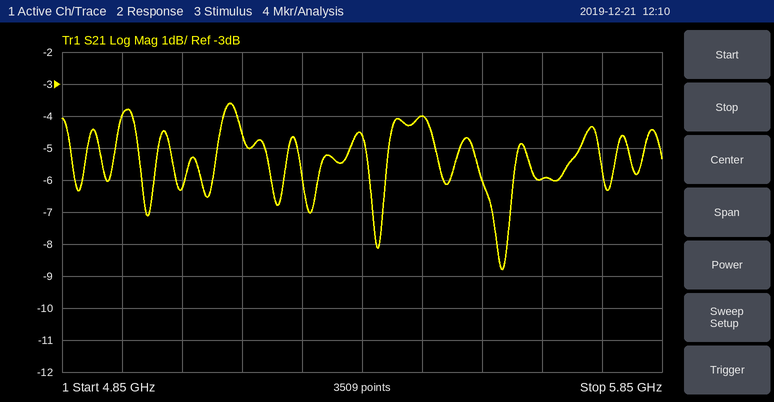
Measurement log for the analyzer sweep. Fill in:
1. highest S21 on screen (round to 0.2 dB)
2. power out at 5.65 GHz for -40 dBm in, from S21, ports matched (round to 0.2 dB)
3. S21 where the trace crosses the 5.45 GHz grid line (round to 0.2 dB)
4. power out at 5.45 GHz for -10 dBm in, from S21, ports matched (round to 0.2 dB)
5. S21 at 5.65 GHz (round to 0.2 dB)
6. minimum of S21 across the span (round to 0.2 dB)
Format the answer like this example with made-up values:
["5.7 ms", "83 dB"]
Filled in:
["-3.6 dB", "-46.0 dBm", "-4.0 dB", "-14.0 dBm", "-6.0 dB", "-8.8 dB"]
